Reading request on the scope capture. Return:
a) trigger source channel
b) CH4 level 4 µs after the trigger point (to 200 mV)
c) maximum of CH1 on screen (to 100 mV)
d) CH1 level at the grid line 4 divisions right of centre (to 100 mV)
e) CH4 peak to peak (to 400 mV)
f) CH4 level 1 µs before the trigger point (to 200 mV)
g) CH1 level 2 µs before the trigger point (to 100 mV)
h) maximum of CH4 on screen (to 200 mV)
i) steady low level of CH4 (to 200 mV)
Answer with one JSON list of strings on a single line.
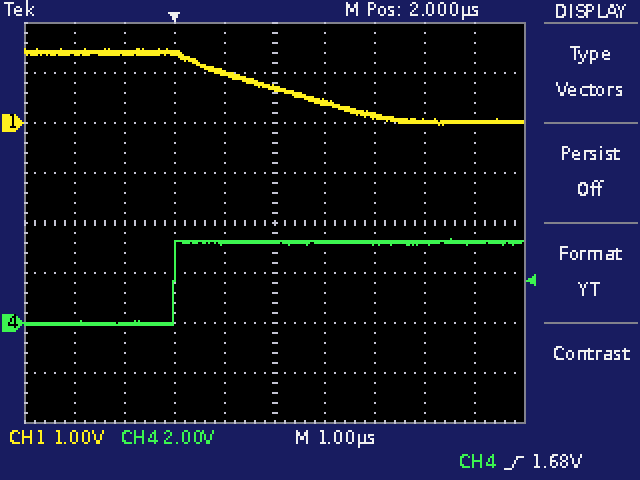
["CH4", "3.2 V", "1.5 V", "0.0 V", "3.6 V", "0.0 V", "1.4 V", "3.4 V", "0.0 V"]
